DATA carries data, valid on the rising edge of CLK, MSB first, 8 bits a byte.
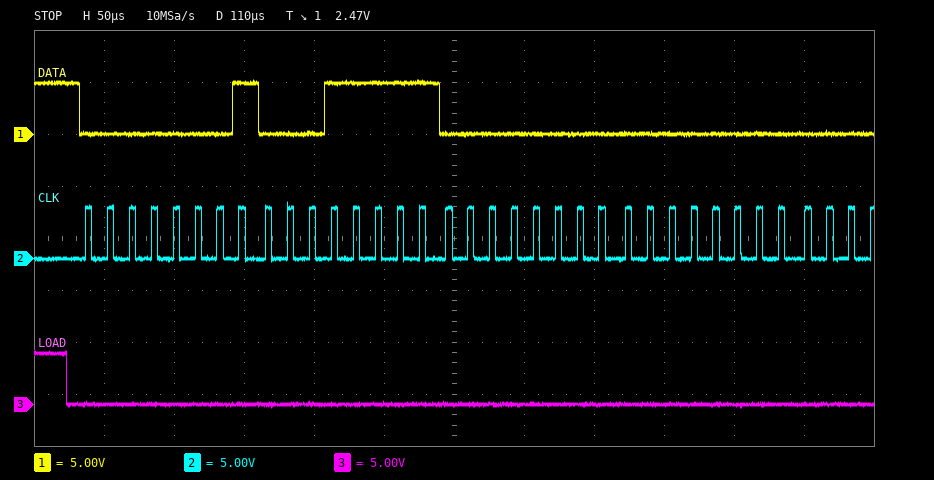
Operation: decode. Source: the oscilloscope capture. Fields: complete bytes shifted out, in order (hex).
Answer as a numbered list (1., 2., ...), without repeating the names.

1. 01 1F 00 00
